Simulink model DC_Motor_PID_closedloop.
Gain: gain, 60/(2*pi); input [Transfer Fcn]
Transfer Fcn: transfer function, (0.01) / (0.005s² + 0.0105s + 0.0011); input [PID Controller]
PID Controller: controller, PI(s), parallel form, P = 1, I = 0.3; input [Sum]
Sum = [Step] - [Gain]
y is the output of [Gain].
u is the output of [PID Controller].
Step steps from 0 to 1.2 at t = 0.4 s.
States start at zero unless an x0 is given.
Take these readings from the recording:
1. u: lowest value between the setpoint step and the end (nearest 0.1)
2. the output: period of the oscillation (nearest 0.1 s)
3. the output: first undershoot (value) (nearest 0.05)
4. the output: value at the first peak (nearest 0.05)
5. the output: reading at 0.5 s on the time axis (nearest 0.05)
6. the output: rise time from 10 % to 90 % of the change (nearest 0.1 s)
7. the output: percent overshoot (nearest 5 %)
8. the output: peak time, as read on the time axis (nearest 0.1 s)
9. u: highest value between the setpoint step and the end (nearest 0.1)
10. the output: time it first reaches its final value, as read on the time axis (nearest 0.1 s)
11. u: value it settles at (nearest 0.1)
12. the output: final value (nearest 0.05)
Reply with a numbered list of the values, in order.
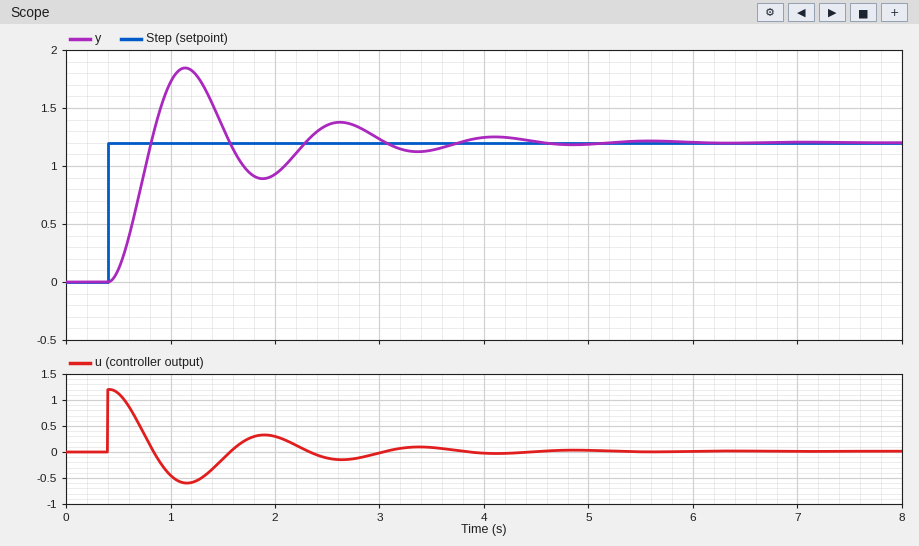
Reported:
1. -0.6
2. 1.5 s
3. 0.90
4. 1.85
5. 0.10
6. 0.3 s
7. 55 %
8. 1.1 s
9. 1.2
10. 0.8 s
11. 0.0
12. 1.20
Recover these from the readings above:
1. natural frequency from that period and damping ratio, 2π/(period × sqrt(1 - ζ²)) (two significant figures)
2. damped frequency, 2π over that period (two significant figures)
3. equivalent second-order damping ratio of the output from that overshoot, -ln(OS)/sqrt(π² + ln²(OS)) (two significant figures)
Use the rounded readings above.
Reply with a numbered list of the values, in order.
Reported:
1. 4.3 rad/s
2. 4.2 rad/s
3. 0.19
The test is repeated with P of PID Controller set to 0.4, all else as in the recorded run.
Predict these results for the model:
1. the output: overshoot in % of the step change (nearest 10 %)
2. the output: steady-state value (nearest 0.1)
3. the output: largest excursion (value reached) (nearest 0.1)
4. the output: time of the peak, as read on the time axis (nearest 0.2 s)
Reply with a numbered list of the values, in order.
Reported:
1. 60 %
2. 1.2
3. 1.9
4. 1.6 s
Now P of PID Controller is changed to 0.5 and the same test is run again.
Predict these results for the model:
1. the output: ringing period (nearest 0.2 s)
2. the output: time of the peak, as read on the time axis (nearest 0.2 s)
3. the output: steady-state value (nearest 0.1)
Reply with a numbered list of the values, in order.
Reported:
1. 2.2 s
2. 1.4 s
3. 1.2
